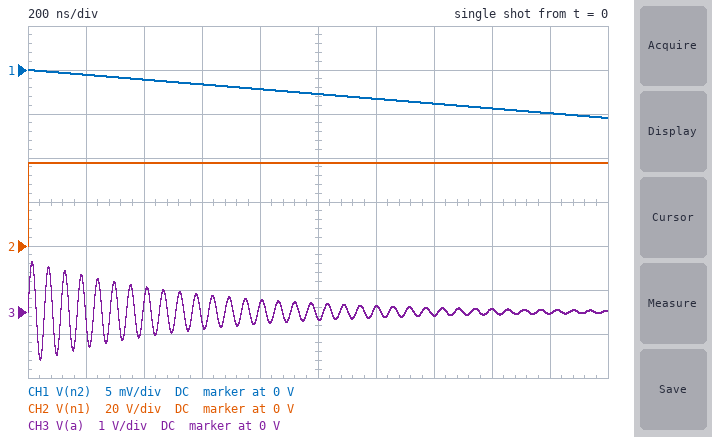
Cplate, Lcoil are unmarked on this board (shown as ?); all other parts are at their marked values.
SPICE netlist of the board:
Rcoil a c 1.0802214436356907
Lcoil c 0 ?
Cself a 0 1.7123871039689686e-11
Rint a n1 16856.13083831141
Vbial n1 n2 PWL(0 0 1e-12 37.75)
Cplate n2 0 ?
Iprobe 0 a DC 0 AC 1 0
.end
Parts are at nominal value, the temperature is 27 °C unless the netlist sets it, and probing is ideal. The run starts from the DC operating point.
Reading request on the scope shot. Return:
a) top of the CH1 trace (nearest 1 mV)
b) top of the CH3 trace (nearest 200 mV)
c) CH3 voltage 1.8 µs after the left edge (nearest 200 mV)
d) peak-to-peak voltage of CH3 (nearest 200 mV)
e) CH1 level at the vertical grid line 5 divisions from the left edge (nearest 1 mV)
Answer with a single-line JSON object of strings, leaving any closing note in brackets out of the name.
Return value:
{"top of the CH1 trace": "0 V", "top of the CH3 trace": "1.2 V", "CH3 voltage 1.8 µs after the left edge": "0 V", "peak-to-peak voltage of CH3": "2.2 V", "CH1 level at the vertical grid line 5 divisions from the left edge": "-3 mV"}
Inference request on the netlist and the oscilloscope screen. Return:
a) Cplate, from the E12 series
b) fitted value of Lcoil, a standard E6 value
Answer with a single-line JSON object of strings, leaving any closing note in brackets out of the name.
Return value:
{"Cplate, from the E12 series": "820 nF", "fitted value of Lcoil, a standard E6 value": "4.7 µH"}
